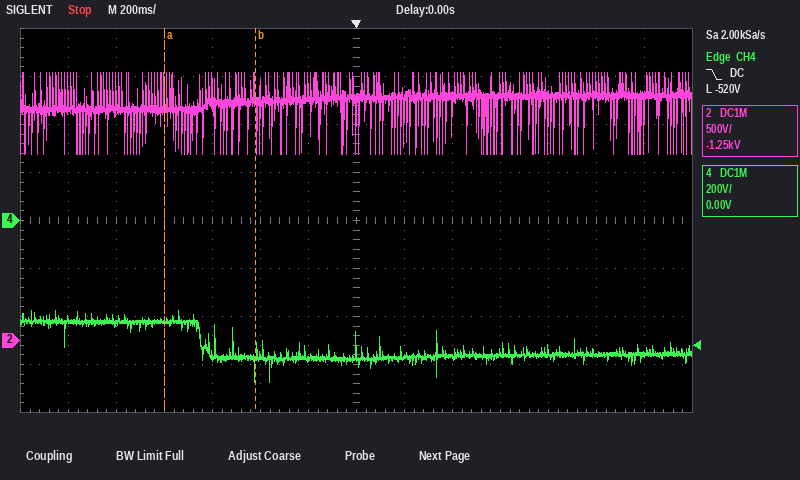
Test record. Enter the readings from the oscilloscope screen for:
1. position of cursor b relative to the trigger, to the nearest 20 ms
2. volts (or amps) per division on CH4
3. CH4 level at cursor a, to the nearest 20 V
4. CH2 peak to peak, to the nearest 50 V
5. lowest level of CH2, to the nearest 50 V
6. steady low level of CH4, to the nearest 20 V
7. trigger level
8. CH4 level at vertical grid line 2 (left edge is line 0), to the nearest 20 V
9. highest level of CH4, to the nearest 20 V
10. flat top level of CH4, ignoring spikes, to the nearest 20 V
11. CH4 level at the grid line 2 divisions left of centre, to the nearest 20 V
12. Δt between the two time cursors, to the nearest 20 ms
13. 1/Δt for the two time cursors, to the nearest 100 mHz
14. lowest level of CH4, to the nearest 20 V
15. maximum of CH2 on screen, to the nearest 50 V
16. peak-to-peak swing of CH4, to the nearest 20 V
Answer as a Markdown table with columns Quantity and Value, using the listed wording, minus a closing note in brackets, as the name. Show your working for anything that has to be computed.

| Quantity | Value |
|---|---|
| position of cursor b relative to the trigger, to the nearest 20 ms | -420 ms |
| volts (or amps) per division on CH4 | 200 V |
| CH4 level at cursor a, to the nearest 20 V | -420 V |
| CH2 peak to peak, to the nearest 50 V | 2.80 kV − (1.95 kV) = 850 V |
| lowest level of CH2, to the nearest 50 V | 1.95 kV |
| steady low level of CH4, to the nearest 20 V | -560 V |
| trigger level | -520 V |
| CH4 level at vertical grid line 2 (left edge is line 0), to the nearest 20 V | -420 V |
| highest level of CH4, to the nearest 20 V | -380 V |
| flat top level of CH4, ignoring spikes, to the nearest 20 V | -420 V |
| CH4 level at the grid line 2 divisions left of centre, to the nearest 20 V | -560 V |
| Δt between the two time cursors, to the nearest 20 ms | 380 ms |
| 1/Δt for the two time cursors, to the nearest 100 mHz | 1 / 380 ms ≈ 2.6 Hz |
| lowest level of CH4, to the nearest 20 V | -680 V |
| maximum of CH2 on screen, to the nearest 50 V | 2.80 kV |
| peak-to-peak swing of CH4, to the nearest 20 V | -380 V − (-680 V) = 300 V |
